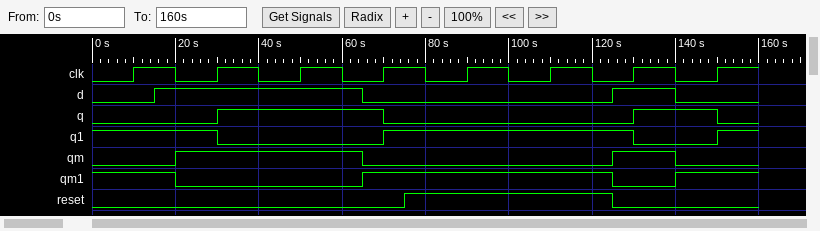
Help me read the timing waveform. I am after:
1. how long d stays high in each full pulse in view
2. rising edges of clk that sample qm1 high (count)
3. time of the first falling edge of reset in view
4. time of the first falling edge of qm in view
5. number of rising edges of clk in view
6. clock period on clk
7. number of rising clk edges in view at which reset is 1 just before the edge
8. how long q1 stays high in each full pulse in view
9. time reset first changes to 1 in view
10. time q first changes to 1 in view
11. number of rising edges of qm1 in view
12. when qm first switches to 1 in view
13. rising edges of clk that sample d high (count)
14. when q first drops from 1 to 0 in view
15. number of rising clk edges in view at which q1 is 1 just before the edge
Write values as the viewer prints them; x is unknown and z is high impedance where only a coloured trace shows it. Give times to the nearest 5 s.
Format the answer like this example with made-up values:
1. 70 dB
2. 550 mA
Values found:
1. 50 s, 15 s
2. 5
3. 125 s
4. 65 s
5. 8
6. 20 s
7. 2
8. 60 s
9. 75 s
10. 30 s
11. 2
12. 20 s
13. 3
14. 70 s
15. 5
